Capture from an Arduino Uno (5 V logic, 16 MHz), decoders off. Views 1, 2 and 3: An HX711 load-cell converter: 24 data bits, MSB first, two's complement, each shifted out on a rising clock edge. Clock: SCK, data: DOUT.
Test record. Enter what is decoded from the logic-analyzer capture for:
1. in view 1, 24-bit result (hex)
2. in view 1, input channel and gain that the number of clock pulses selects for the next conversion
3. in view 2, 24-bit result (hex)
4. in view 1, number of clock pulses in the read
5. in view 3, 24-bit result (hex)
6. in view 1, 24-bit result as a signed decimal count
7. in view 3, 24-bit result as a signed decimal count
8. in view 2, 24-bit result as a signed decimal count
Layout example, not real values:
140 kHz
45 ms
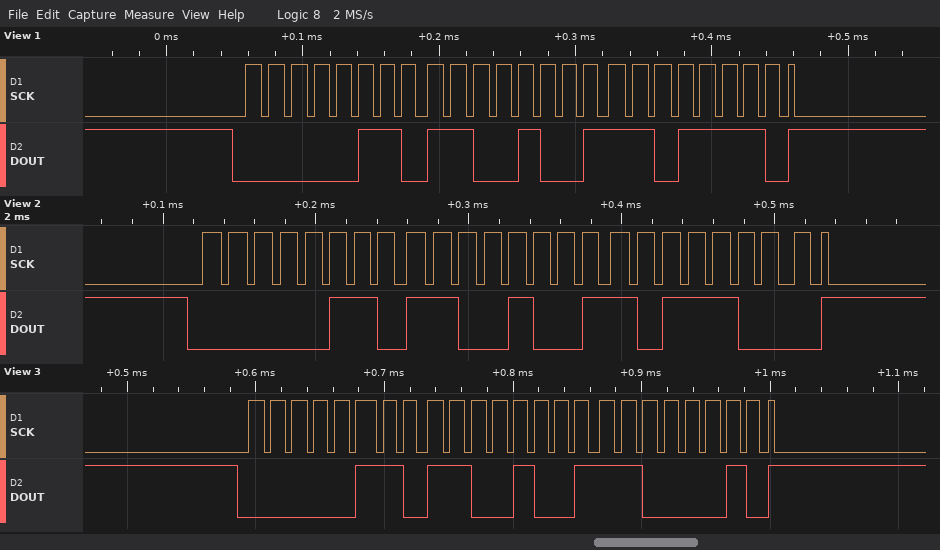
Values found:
0x06C9DE
channel A, gain 128
0x06C9B8
25
0x06C9C2
444894
444866
444856
